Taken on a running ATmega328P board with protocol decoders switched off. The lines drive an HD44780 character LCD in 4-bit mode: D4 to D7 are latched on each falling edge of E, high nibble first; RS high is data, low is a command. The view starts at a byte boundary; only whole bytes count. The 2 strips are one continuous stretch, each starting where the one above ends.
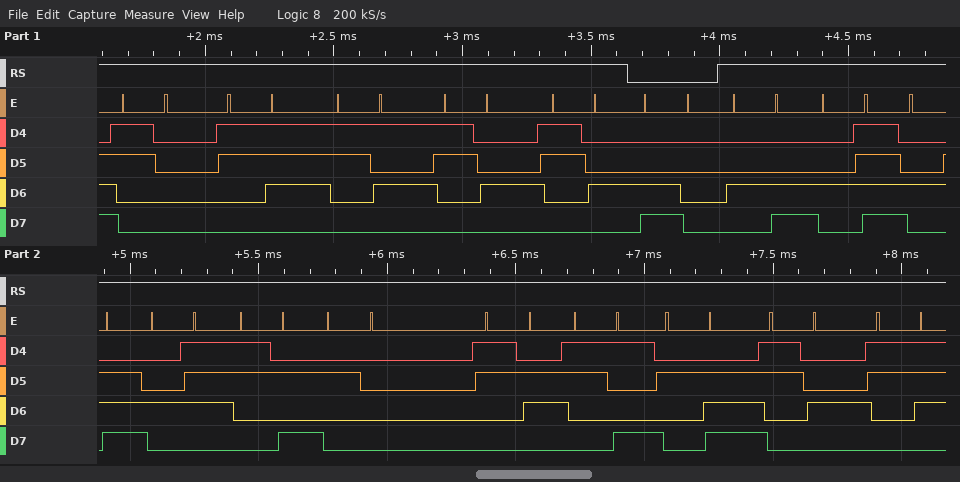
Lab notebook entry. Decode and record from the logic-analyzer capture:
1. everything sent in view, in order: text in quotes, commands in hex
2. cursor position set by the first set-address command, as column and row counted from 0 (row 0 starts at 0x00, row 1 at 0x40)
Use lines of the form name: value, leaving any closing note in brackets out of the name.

everything sent in view, in order: text in quotes, commands in hex: "07544" 0xC0 "LONG: 69.47"
cursor position set by the first set-address command, as column and row counted from 0: column 0, row 1
